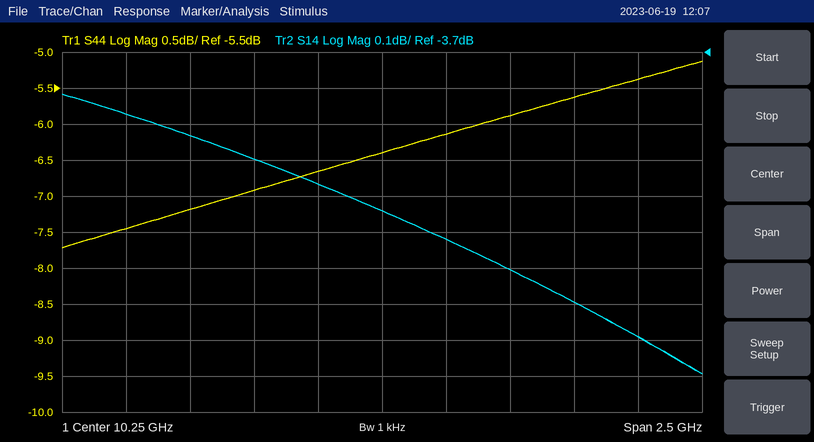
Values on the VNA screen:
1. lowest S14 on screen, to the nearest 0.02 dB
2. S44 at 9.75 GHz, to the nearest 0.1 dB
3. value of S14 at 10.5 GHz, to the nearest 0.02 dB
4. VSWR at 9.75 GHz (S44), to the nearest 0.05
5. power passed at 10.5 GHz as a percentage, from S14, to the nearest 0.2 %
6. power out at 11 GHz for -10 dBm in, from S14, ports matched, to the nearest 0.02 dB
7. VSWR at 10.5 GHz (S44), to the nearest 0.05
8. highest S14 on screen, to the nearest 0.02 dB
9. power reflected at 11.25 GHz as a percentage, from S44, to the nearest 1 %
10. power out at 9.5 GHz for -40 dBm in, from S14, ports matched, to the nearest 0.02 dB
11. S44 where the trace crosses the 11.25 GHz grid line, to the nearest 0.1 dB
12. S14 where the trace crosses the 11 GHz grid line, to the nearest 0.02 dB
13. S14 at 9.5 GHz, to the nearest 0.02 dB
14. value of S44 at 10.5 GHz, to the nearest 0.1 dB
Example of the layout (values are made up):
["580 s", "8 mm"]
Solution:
["-4.60 dB", "-6.9 dB", "-4.22 dB", "2.65", "37.8 %", "-14.40 dBm", "2.95", "-3.82 dB", "29 %", "-43.94 dBm", "-5.4 dB", "-4.40 dB", "-3.94 dB", "-6.1 dB"]
